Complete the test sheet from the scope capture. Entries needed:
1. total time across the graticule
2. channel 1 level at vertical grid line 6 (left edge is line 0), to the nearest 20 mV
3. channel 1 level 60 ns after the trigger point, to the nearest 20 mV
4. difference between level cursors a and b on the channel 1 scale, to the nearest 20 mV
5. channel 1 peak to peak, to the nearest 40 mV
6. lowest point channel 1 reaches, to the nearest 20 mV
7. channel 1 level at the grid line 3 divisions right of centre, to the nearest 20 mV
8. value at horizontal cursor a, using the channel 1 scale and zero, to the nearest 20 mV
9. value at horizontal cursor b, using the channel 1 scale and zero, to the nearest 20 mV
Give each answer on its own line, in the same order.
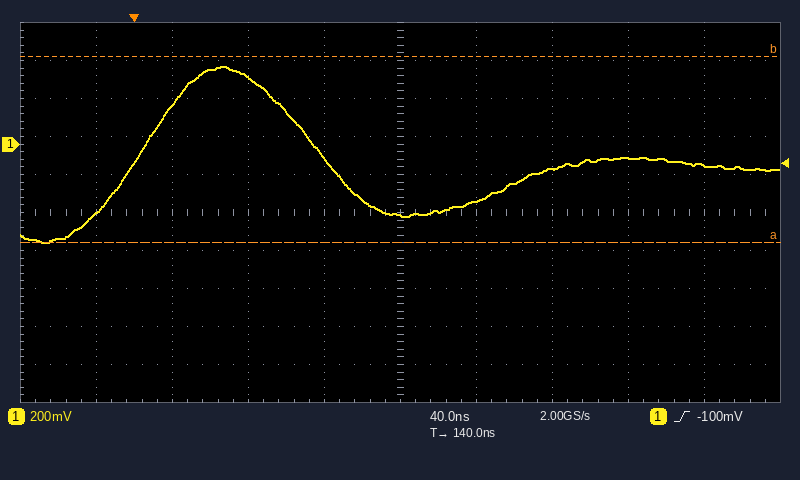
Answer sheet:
400 ns
-300 mV
360 mV
980 mV
920 mV
-520 mV
-80 mV
-520 mV
460 mV
